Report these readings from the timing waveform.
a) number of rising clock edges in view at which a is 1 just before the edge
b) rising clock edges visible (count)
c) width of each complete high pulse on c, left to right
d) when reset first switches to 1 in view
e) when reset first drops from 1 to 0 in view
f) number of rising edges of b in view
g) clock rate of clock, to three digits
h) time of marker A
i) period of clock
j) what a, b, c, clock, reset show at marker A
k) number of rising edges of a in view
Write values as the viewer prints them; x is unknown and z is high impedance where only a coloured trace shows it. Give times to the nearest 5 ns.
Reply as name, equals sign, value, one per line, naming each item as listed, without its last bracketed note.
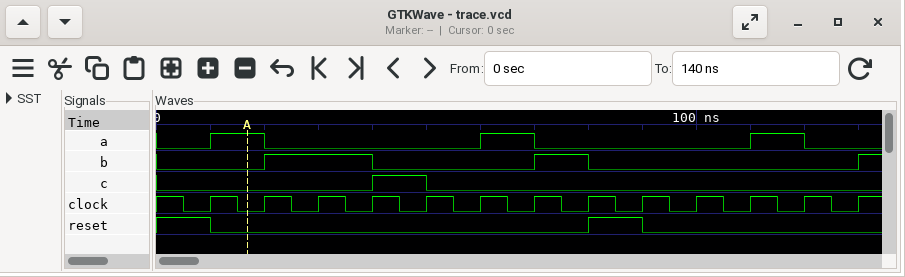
number of rising clock edges in view at which a is 1 just before the edge = 3
rising clock edges visible = 13
width of each complete high pulse on c, left to right = 10 ns
when reset first switches to 1 in view = 80 ns
when reset first drops from 1 to 0 in view = 10 ns
number of rising edges of b in view = 3
clock rate of clock, to three digits = 100 MHz
time of marker A = 15 ns
period of clock = 10 ns
what a, b, c, clock, reset show at marker A = a=1, b=0, c=0, clock=0, reset=0
number of rising edges of a in view = 3
